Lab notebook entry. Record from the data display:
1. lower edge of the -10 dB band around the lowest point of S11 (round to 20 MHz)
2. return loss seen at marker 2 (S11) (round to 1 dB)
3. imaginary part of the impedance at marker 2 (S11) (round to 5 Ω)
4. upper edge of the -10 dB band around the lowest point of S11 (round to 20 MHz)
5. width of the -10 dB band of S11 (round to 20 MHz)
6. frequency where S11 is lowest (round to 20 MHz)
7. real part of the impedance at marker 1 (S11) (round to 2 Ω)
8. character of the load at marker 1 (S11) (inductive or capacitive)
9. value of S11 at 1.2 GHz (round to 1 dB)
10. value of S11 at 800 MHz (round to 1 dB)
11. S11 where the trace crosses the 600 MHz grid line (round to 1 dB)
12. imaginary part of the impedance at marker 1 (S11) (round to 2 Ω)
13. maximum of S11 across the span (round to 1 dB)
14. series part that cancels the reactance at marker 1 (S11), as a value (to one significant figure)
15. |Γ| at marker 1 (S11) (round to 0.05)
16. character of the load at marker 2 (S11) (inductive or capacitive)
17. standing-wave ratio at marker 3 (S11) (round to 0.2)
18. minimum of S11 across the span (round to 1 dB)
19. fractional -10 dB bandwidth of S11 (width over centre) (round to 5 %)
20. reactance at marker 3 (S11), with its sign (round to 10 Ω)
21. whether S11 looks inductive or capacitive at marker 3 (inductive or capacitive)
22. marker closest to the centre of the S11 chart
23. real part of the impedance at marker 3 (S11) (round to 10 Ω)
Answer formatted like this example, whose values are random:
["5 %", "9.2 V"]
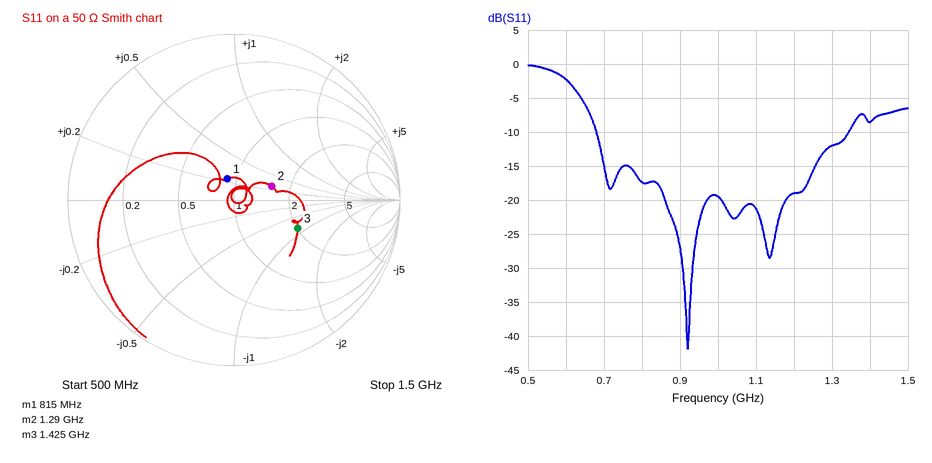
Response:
["680 MHz", "12 dB", "+15 Ω", "1.34 GHz", "660 MHz", "920 MHz", "44 Ω", "inductive", "-19 dB", "-17 dB", "-2 dB", "+12 Ω", "0 dB", "20 pF", "0.15", "inductive", "2.4", "-42 dB", "65 %", "-40 Ω", "capacitive", "marker 1", "100 Ω"]
